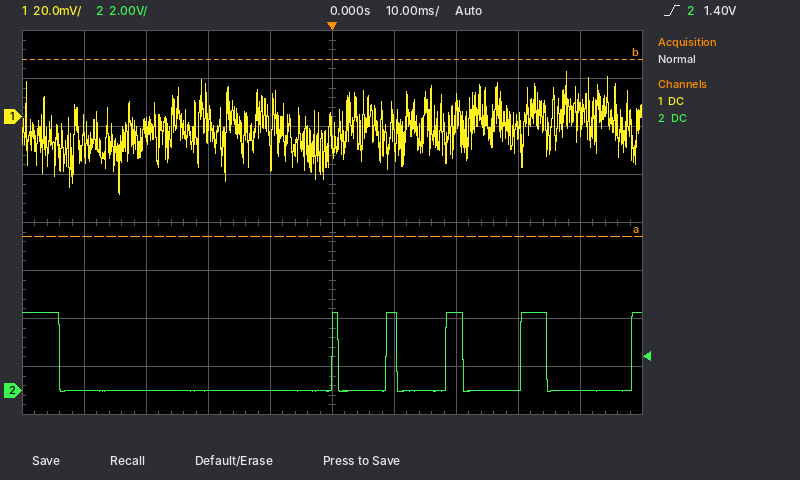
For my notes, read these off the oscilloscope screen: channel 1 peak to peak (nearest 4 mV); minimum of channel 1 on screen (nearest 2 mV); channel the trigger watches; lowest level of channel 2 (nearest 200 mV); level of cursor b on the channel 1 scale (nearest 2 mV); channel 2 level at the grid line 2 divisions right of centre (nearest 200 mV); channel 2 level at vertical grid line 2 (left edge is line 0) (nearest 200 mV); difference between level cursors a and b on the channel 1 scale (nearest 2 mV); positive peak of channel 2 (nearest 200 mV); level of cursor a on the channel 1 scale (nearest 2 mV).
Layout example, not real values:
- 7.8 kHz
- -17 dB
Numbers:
- 52 mV
- -32 mV
- channel 2
- 0.0 V
- 24 mV
- 3.2 V
- 0.0 V
- 74 mV
- 3.2 V
- -50 mV
